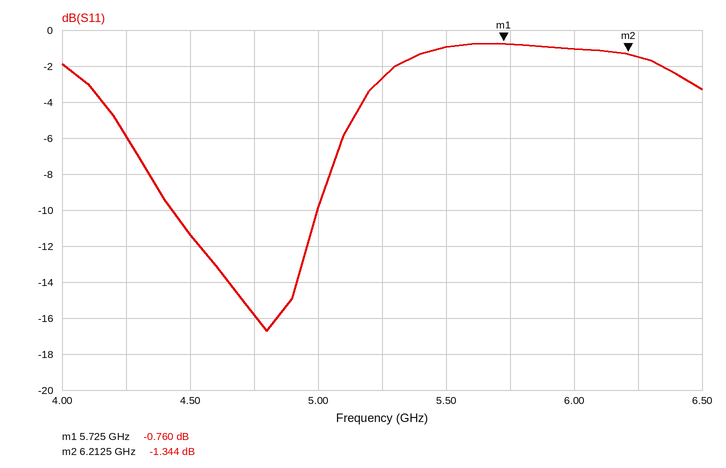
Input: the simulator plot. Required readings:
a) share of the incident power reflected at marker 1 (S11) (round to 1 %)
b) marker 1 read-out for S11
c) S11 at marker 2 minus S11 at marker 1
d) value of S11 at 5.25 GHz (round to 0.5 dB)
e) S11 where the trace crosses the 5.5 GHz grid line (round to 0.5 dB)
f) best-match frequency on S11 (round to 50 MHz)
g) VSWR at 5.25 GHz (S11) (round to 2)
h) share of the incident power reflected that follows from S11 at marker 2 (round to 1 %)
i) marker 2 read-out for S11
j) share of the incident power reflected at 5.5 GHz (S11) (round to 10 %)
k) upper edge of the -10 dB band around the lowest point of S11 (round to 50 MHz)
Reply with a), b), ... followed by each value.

a) 84 %
b) -0.760 dB
c) -0.584 dB
d) -2.5 dB
e) -1.0 dB
f) 4.80 GHz
g) 6
h) 73 %
i) -1.344 dB
j) 80 %
k) 5.00 GHz
